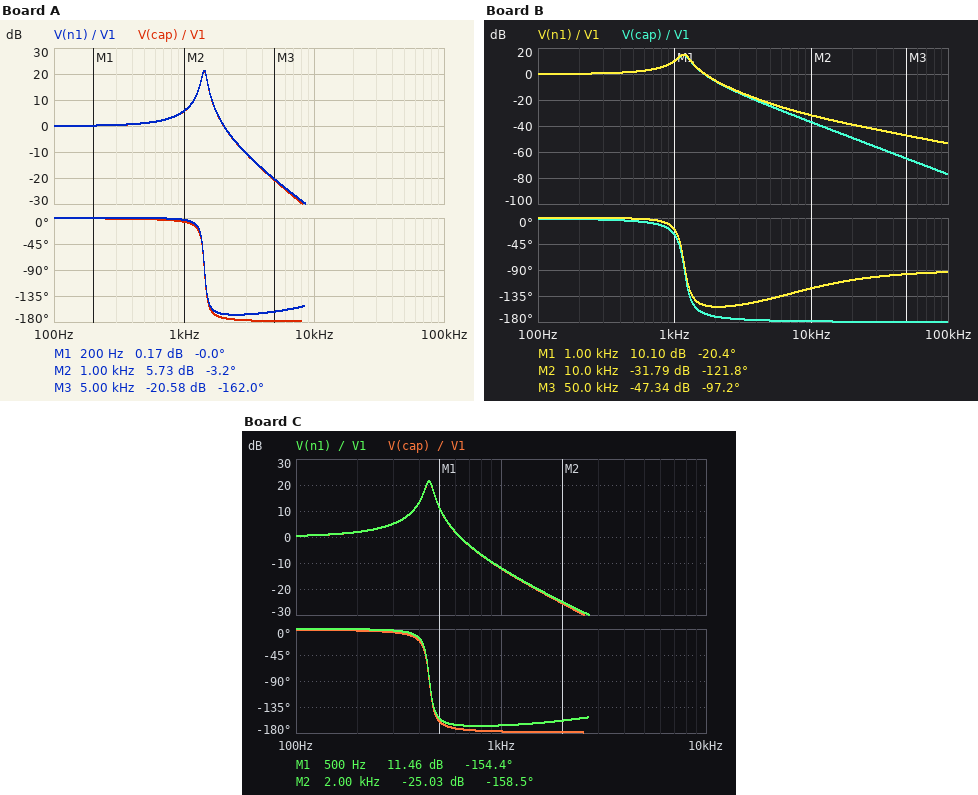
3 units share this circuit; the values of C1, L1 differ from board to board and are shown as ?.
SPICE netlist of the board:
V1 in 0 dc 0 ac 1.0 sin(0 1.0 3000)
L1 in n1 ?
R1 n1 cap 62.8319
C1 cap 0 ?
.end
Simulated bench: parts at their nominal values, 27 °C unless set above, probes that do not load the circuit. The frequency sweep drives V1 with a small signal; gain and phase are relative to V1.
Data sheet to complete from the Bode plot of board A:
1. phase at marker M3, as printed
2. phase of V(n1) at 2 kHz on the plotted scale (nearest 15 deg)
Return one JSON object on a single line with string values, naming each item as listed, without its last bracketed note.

{"phase at marker M3, as printed": "-162.0 deg", "phase of V(n1) at 2 kHz on the plotted scale": "-165 deg"}
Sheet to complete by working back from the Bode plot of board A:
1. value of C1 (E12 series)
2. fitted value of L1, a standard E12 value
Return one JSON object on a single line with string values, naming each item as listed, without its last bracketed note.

{"value of C1": "150 nF", "fitted value of L1, a standard E12 value": "82 mH"}
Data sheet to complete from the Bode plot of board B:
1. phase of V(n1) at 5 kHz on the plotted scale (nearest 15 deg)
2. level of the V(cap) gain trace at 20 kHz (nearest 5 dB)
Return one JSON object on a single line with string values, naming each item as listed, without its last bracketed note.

{"phase of V(n1) at 5 kHz on the plotted scale": "-135 deg", "level of the V(cap) gain trace at 20 kHz": "-50 dB"}
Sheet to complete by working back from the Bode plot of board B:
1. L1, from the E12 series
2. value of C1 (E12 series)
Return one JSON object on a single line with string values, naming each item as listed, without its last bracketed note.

{"L1, from the E12 series": "47 mH", "value of C1": "390 nF"}
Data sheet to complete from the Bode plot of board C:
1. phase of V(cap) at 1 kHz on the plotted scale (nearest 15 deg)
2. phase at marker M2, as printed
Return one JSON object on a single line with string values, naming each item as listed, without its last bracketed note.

{"phase of V(cap) at 1 kHz on the plotted scale": "-180 deg", "phase at marker M2, as printed": "-158.5 deg"}
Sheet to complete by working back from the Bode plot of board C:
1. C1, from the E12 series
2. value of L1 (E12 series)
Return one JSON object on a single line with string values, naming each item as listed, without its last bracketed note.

{"C1, from the E12 series": "470 nF", "value of L1": "270 mH"}
